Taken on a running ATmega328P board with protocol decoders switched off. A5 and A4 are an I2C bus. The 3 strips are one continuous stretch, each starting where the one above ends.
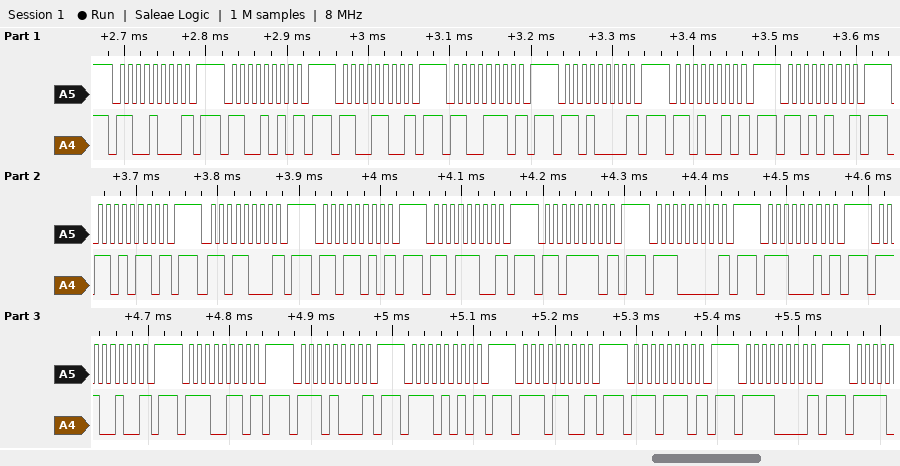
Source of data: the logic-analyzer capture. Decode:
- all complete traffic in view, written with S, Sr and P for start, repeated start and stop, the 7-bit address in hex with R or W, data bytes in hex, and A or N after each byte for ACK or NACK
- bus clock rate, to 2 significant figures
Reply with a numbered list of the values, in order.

1. S 64W N P S 65W N P S 66W N P S 67W N P S 68W N P S 69W N P S 6AW N P S 6BW N P S 6CW N P S 6DW N P S 6EW N P S 6FW N P S 70W N P S 71W N P S 72W N P S 73W N P S 74W N P S 75W N P S 76W N P S 77W N P S 78W N P
2. 100 kHz
